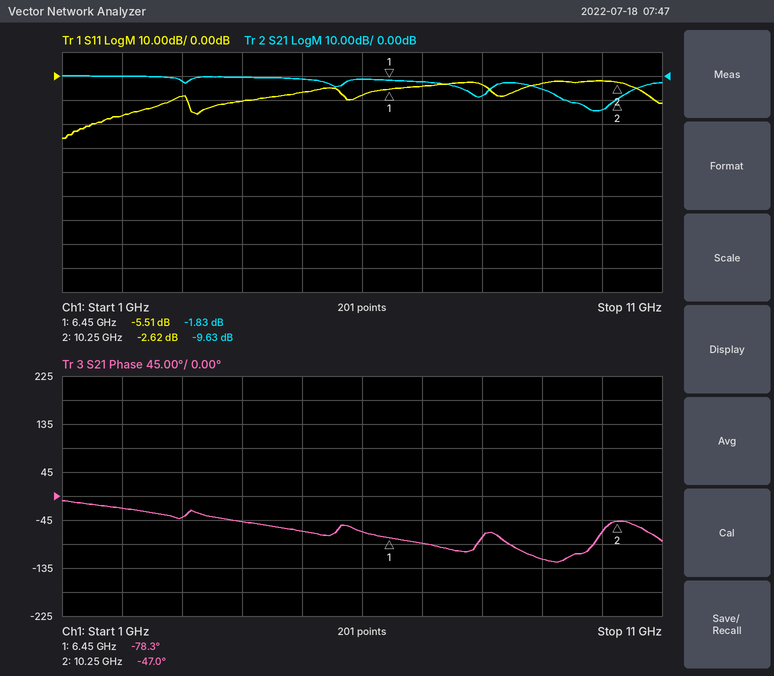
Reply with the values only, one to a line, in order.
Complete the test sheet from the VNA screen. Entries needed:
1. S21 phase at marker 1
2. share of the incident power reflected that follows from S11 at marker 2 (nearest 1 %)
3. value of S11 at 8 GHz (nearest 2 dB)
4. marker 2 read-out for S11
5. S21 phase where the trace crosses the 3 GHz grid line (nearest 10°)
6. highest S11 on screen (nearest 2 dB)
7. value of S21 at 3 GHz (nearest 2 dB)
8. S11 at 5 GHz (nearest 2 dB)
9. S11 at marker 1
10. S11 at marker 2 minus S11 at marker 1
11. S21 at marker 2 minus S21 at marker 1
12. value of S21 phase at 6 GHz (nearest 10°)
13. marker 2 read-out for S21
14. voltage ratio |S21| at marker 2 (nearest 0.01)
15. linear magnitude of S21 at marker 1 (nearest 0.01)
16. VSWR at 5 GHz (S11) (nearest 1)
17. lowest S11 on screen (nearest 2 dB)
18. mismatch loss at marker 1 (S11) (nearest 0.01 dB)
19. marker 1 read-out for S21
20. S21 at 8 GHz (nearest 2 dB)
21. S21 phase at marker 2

-78.3°
55 %
-4 dB
-2.62 dB
-40°
-2 dB
-2 dB
-6 dB
-5.51 dB
2.89 dB
-7.80 dB
-70°
-9.63 dB
0.33
0.81
3
-26 dB
1.43 dB
-1.83 dB
-8 dB
-47.0°
